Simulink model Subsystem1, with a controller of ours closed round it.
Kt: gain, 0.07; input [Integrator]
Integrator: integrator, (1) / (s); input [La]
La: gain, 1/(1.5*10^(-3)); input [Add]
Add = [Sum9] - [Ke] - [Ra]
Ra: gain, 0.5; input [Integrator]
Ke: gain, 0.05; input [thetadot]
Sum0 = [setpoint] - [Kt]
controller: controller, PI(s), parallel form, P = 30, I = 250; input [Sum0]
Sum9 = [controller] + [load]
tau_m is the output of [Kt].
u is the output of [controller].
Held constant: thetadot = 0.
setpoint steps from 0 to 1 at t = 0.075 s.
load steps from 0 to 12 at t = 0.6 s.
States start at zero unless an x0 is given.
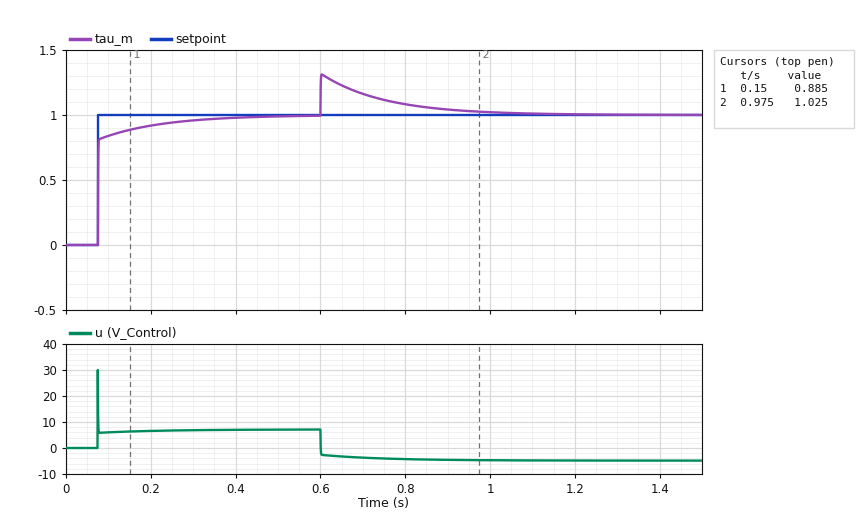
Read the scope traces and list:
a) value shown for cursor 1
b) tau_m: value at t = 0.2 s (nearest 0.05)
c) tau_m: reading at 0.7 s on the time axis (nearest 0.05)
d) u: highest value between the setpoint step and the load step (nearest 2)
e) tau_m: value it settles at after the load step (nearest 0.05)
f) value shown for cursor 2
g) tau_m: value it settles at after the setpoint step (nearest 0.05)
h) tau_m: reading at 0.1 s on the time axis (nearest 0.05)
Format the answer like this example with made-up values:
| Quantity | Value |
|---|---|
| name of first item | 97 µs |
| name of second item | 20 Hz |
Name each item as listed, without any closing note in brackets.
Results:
| Quantity | Value |
|---|---|
| value shown for cursor 1 | 0.885 |
| tau_m: value at t = 0.2 s | 0.90 |
| tau_m: reading at 0.7 s on the time axis | 1.15 |
| u: highest value between the setpoint step and the load step | 30 |
| tau_m: value it settles at after the load step | 1.00 |
| value shown for cursor 2 | 1.025 |
| tau_m: value it settles at after the setpoint step | 1.00 |
| tau_m: reading at 0.1 s on the time axis | 0.85 |
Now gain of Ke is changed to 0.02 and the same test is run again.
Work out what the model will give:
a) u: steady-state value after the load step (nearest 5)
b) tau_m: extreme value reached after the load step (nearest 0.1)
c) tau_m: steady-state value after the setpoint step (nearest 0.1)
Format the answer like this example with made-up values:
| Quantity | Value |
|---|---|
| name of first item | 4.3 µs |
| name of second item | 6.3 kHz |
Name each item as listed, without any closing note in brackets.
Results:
| Quantity | Value |
|---|---|
| u: steady-state value after the load step | -5 |
| tau_m: extreme value reached after the load step | 1.3 |
| tau_m: steady-state value after the setpoint step | 1.0 |
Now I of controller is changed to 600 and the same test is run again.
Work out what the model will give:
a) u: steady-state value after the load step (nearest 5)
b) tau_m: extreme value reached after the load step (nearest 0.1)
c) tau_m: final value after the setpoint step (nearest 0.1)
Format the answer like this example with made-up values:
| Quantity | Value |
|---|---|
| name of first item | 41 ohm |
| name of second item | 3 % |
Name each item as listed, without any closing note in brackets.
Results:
| Quantity | Value |
|---|---|
| u: steady-state value after the load step | -5 |
| tau_m: extreme value reached after the load step | 1.3 |
| tau_m: final value after the setpoint step | 1.0 |
